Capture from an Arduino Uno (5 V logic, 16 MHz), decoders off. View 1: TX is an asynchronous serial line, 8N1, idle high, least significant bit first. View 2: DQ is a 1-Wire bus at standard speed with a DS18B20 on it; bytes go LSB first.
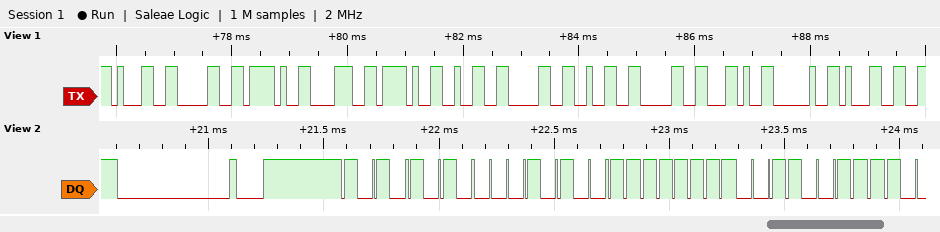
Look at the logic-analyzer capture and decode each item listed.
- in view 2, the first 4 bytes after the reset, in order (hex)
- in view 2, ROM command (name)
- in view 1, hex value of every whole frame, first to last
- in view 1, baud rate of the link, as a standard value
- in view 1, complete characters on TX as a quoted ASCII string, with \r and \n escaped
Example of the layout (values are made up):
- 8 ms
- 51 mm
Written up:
- 55 28 FF CC
- Match ROM
- 31 30 2F 38 2F 32 30 32 30 2C 20 31
- 9600 baud
- "10/8/2020, 1"
